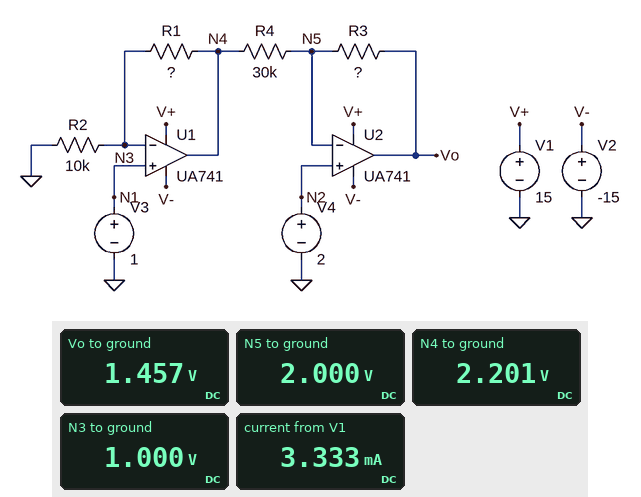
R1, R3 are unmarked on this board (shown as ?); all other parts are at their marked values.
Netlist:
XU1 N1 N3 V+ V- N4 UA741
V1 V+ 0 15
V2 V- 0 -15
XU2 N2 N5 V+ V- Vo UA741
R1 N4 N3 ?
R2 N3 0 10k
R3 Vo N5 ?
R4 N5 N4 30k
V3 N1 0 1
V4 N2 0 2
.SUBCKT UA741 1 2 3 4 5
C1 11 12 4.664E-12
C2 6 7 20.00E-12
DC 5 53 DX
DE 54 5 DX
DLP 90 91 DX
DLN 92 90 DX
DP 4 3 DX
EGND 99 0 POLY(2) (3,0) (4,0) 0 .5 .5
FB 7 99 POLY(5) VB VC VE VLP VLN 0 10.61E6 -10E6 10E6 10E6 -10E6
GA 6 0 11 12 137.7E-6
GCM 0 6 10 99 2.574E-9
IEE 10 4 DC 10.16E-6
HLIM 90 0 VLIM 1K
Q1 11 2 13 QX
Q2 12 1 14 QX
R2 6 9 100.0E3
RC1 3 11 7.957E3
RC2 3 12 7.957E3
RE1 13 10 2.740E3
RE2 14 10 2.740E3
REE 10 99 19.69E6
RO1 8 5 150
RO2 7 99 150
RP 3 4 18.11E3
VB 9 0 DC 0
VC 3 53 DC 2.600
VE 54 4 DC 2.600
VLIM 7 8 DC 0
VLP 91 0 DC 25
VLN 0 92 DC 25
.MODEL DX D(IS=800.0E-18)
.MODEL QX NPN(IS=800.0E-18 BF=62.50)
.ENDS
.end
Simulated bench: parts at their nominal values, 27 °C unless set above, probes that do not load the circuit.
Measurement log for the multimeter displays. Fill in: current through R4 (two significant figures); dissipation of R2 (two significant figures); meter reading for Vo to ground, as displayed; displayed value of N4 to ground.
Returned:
6.7 µA
100 µW
1.457 V
2.201 V
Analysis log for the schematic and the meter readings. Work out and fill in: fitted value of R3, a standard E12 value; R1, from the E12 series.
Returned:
82 kΩ
12 kΩ
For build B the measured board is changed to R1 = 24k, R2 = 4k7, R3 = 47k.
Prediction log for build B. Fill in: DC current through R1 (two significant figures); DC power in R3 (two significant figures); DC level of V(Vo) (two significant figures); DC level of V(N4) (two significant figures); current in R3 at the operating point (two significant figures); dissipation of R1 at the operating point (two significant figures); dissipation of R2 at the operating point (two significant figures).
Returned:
210 µA
880 µW
-4.4 V
6.1 V
140 µA
1.1 mW
210 µW
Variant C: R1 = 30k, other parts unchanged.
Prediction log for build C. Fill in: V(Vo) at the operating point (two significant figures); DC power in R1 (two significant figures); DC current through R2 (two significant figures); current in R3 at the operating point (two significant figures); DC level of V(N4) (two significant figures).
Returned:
-3.5 V
300 µW
100 µA
67 µA
4.0 V
